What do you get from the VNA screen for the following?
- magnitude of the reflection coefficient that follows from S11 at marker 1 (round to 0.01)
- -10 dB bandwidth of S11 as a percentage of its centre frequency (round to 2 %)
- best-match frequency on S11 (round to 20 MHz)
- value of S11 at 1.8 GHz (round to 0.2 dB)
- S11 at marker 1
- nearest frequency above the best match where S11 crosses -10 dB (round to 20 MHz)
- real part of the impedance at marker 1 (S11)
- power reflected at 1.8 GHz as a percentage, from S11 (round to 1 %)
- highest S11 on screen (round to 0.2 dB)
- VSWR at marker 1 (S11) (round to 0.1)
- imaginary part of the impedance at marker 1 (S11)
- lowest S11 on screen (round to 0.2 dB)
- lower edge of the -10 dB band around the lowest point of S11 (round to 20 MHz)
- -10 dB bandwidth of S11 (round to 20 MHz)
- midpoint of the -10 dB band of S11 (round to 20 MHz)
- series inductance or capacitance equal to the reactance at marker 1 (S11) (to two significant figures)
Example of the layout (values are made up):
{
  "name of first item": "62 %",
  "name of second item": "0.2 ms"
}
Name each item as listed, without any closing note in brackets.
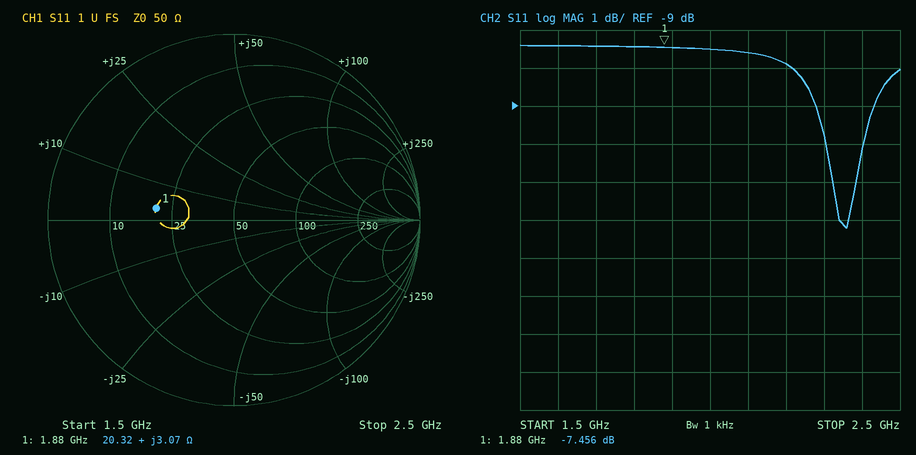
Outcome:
{
  "magnitude of the reflection coefficient that follows from S11 at marker 1": "0.42",
  "-10 dB bandwidth of S11 as a percentage of its centre frequency": "4 %",
  "best-match frequency on S11": "2.36 GHz",
  "value of S11 at 1.8 GHz": "-7.4 dB",
  "S11 at marker 1": "-7.456 dB",
  "nearest frequency above the best match where S11 crosses -10 dB": "2.40 GHz",
  "real part of the impedance at marker 1": "20.32 Ω",
  "power reflected at 1.8 GHz as a percentage, from S11": "18 %",
  "highest S11 on screen": "-7.4 dB",
  "VSWR at marker 1 (S11)": "2.5",
  "imaginary part of the impedance at marker 1": "+3.07 Ω",
  "lowest S11 on screen": "-12.2 dB",
  "lower edge of the -10 dB band around the lowest point of S11": "2.30 GHz",
  "-10 dB bandwidth of S11": "100 MHz",
  "midpoint of the -10 dB band of S11": "2.36 GHz",
  "series inductance or capacitance equal to the reactance at marker 1 (S11)": "260 pH"
}
